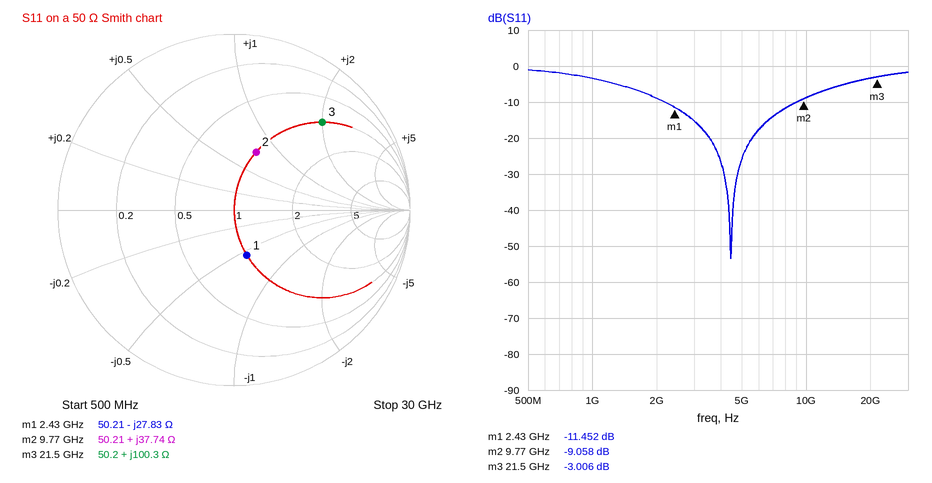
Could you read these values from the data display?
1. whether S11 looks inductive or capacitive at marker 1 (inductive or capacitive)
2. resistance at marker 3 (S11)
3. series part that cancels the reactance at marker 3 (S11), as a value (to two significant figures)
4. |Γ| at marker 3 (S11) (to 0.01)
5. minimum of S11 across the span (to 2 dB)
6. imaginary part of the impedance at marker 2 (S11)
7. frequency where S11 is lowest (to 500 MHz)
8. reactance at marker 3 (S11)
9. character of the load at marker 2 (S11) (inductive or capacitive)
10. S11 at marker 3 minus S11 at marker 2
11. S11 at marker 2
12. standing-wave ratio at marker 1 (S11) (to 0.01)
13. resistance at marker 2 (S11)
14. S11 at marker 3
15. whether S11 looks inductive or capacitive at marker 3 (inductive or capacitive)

capacitive
50.2 Ω
74 fF
0.71
-54 dB
+37.74 Ω
4.5 GHz
+100.3 Ω
inductive
6.052 dB
-9.058 dB
1.73
50.21 Ω
-3.006 dB
inductive
